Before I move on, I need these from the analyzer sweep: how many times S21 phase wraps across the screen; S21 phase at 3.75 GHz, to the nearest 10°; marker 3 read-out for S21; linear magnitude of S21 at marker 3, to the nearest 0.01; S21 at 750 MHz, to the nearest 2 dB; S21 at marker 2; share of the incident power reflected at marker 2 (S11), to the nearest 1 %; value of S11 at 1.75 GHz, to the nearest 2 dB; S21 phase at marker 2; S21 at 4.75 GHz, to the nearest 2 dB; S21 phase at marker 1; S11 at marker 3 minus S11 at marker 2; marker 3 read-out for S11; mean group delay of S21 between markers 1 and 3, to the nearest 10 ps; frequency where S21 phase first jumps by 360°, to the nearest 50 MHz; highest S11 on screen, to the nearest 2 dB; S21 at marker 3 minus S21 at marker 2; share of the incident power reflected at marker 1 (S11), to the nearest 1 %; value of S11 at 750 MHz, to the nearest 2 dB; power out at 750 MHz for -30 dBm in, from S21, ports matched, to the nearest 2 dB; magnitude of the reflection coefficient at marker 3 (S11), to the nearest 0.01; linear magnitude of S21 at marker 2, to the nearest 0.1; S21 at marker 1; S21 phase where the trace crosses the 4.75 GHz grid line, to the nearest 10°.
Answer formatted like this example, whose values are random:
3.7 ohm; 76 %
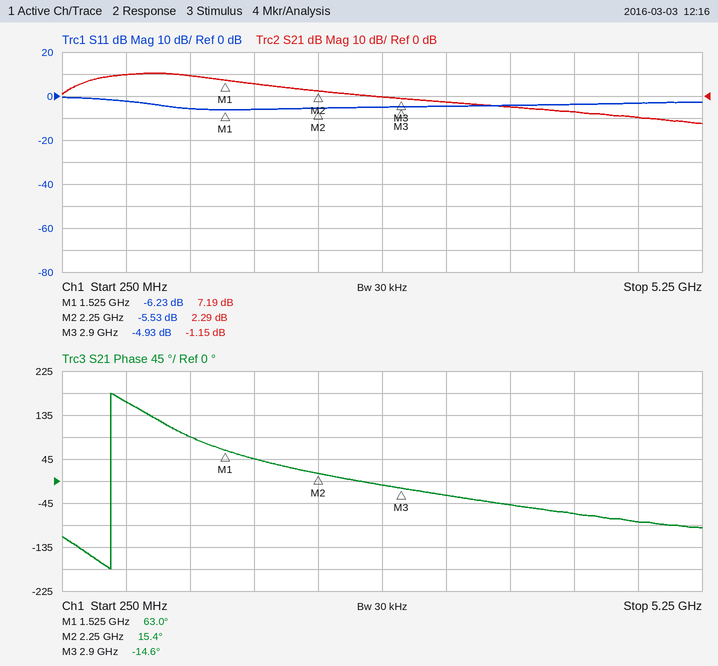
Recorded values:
1; -50°; -1.15 dB; 0.88; 10 dB; 2.29 dB; 28 %; -6 dB; 15.4°; -10 dB; 63.0°; 0.60 dB; -4.93 dB; 160 ps; 650 MHz; 0 dB; -3.44 dB; 24 %; -2 dB; -20 dBm; 0.57; 1.3; 7.19 dB; -80°
